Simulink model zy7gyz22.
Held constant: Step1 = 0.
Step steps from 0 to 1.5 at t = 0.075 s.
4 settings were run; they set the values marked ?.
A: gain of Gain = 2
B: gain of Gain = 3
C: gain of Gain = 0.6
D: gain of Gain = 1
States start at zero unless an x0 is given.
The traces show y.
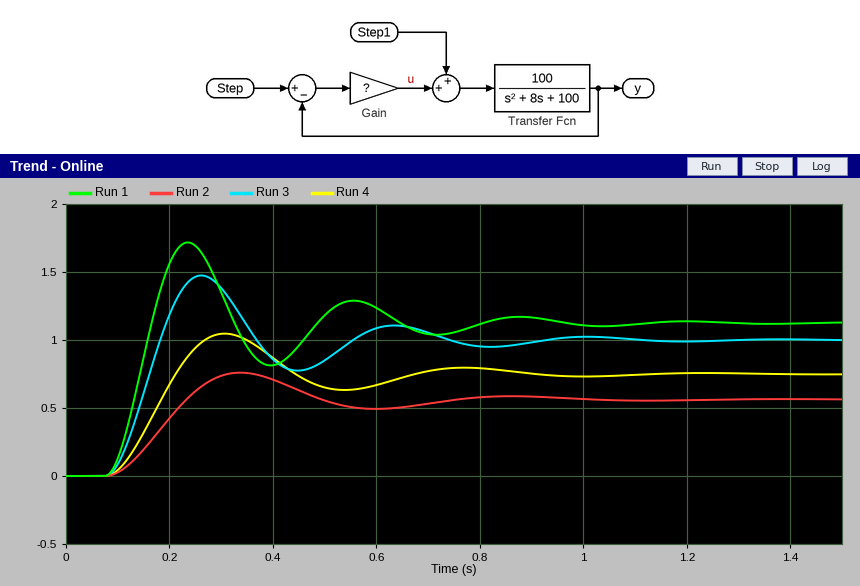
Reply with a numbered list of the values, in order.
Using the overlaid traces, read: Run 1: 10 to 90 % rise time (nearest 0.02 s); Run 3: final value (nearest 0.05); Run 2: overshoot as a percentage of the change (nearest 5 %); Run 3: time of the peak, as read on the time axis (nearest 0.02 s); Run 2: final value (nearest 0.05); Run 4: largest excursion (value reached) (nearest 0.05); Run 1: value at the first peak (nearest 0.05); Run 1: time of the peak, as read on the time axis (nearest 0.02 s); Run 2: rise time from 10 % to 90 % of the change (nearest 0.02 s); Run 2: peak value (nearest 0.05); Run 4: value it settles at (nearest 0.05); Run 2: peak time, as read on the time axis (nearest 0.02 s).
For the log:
1. 0.06 s
2. 1.00
3. 35 %
4. 0.26 s
5. 0.55
6. 1.05
7. 1.70
8. 0.24 s
9. 0.10 s
10. 0.75
11. 0.75
12. 0.34 s
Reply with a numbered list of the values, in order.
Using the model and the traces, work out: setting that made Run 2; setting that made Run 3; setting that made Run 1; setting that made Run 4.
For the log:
1. C
2. A
3. B
4. D
